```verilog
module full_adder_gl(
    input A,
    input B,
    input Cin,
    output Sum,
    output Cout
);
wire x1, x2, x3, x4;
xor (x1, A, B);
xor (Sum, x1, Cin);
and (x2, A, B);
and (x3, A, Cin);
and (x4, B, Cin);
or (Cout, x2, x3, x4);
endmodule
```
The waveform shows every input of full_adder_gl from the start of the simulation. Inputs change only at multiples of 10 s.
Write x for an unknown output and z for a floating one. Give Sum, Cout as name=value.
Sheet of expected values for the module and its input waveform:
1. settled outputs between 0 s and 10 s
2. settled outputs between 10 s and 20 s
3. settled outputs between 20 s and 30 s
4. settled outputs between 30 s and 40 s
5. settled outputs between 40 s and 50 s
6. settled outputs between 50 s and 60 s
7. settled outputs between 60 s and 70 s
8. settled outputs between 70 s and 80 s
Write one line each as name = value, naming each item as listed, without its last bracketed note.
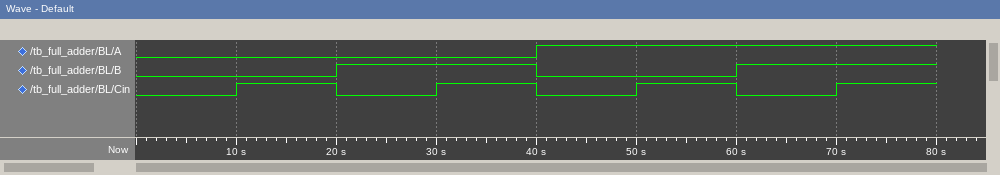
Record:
settled outputs between 0 s and 10 s = Sum=0, Cout=0
settled outputs between 10 s and 20 s = Sum=1, Cout=0
settled outputs between 20 s and 30 s = Sum=1, Cout=0
settled outputs between 30 s and 40 s = Sum=0, Cout=1
settled outputs between 40 s and 50 s = Sum=1, Cout=0
settled outputs between 50 s and 60 s = Sum=0, Cout=1
settled outputs between 60 s and 70 s = Sum=0, Cout=1
settled outputs between 70 s and 80 s = Sum=1, Cout=1
